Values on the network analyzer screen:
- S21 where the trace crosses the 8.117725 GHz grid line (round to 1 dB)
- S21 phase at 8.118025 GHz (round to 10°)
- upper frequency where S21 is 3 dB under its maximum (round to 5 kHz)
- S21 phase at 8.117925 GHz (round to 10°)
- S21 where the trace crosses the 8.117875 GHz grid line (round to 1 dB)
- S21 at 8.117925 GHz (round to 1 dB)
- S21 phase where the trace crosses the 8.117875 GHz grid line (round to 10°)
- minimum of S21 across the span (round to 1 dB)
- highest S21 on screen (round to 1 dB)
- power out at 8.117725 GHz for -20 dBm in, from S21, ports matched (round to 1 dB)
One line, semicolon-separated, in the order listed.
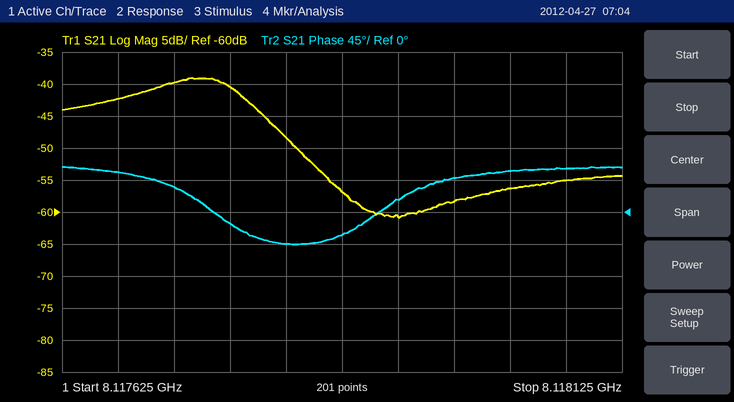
-40 dB; 60°; 8.117785 GHz; 20°; -57 dB; -61 dB; -30°; -61 dB; -39 dB; -60 dBm
